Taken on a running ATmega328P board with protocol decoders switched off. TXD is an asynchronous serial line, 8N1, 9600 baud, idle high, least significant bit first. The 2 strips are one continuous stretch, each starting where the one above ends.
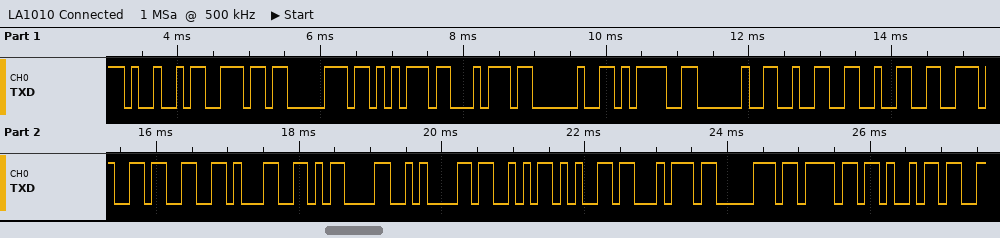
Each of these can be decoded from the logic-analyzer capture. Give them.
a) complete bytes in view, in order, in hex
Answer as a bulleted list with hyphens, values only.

- 0x49 0x6E 0x70 0x75 0x74 0x20 0x3D 0x20 0x32 0x32 0x2E 0x33 0x31 0x0D 0x0A 0x53 0x65 0x74 0x70 0x6F 0x69
